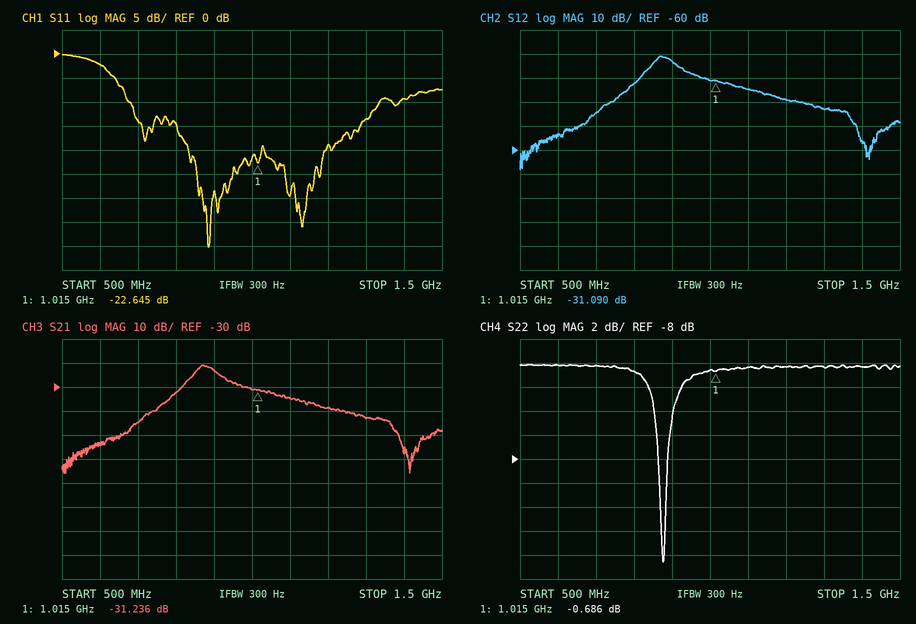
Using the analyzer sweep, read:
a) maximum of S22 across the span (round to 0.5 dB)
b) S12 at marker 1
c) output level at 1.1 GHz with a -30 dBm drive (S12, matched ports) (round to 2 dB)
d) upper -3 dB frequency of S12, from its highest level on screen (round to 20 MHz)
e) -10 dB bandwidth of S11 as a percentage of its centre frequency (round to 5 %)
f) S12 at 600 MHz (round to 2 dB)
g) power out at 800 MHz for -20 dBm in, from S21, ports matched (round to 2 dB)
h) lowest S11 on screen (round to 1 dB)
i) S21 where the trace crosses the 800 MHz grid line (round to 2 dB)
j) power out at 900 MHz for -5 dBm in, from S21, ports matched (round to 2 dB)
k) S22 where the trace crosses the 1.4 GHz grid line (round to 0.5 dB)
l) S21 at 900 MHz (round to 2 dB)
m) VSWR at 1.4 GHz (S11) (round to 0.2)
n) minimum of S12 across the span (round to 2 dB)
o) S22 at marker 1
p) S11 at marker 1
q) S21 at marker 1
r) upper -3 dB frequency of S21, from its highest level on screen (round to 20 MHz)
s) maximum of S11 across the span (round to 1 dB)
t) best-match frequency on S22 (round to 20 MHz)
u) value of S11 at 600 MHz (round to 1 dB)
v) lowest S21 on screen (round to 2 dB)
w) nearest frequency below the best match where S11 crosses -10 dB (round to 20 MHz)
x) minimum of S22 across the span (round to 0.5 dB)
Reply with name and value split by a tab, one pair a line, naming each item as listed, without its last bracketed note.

maximum of S22 across the span	0.0 dB
S12 at marker 1	-31.090 dB
output level at 1.1 GHz with a -30 dBm drive (S12, matched ports)	-64 dBm
upper -3 dB frequency of S12, from its highest level on screen	900 MHz
-10 dB bandwidth of S11 as a percentage of its centre frequency	65 %
S12 at 600 MHz	-54 dB
power out at 800 MHz for -20 dBm in, from S21, ports matched	-52 dBm
lowest S11 on screen	-40 dB
S21 where the trace crosses the 800 MHz grid line	-32 dB
power out at 900 MHz for -5 dBm in, from S21, ports matched	-28 dBm
S22 where the trace crosses the 1.4 GHz grid line	-0.5 dB
S21 at 900 MHz	-24 dB
VSWR at 1.4 GHz (S11)	2.0
minimum of S12 across the span	-68 dB
S22 at marker 1	-0.686 dB
S11 at marker 1	-22.645 dB
S21 at marker 1	-31.236 dB
upper -3 dB frequency of S21, from its highest level on screen	900 MHz
maximum of S11 across the span	0 dB
best-match frequency on S22	880 MHz
value of S11 at 600 MHz	-2 dB
lowest S21 on screen	-66 dB
nearest frequency below the best match where S11 crosses -10 dB	680 MHz
minimum of S22 across the span	-16.5 dB
